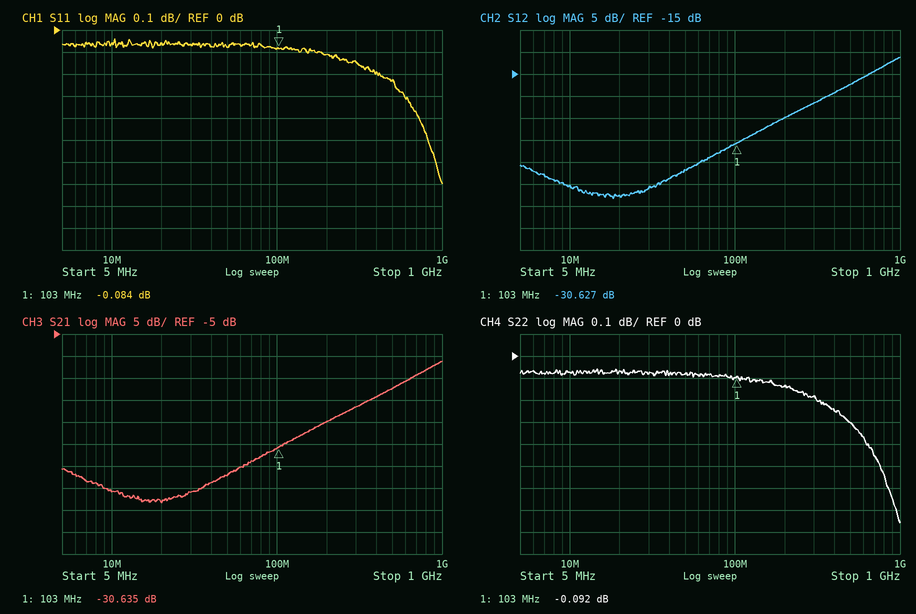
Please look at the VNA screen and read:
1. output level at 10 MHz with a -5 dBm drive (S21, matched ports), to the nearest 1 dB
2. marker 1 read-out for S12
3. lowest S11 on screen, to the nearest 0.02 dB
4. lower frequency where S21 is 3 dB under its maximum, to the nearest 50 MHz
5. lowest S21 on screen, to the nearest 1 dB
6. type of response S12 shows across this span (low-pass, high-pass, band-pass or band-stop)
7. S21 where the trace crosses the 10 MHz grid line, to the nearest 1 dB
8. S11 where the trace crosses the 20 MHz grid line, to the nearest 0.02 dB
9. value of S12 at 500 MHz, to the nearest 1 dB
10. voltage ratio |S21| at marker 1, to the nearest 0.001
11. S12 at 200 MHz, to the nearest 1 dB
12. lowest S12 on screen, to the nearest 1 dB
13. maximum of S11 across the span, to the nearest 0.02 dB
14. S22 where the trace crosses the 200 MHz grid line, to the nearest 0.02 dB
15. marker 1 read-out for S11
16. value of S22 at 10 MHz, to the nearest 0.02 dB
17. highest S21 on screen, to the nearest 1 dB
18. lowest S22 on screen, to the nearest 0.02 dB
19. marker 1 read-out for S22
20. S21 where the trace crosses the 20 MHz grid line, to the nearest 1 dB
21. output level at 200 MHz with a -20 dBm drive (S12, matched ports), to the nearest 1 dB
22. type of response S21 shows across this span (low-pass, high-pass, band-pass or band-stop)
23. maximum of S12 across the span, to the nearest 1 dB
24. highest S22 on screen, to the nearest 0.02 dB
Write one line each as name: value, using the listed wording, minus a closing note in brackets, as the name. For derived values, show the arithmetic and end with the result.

output level at 10 MHz with a -5 dBm drive (S21, matched ports), to the nearest 1 dB: -5 dBm + (-41 dB) = -46 dBm
marker 1 read-out for S12: -30.627 dB
lowest S11 on screen, to the nearest 0.02 dB: -0.70 dB
lower frequency where S21 is 3 dB under its maximum, to the nearest 50 MHz: 700 MHz
lowest S21 on screen, to the nearest 1 dB: -43 dB
type of response S12 shows across this span: high-pass
S21 where the trace crosses the 10 MHz grid line, to the nearest 1 dB: -41 dB
S11 where the trace crosses the 20 MHz grid line, to the nearest 0.02 dB: -0.06 dB
value of S12 at 500 MHz, to the nearest 1 dB: -17 dB
voltage ratio |S21| at marker 1, to the nearest 0.001: 10^(-30.635/20) ≈ 0.029
S12 at 200 MHz, to the nearest 1 dB: -25 dB
lowest S12 on screen, to the nearest 1 dB: -43 dB
maximum of S11 across the span, to the nearest 0.02 dB: -0.04 dB
S22 where the trace crosses the 200 MHz grid line, to the nearest 0.02 dB: -0.14 dB
marker 1 read-out for S11: -0.084 dB
value of S22 at 10 MHz, to the nearest 0.02 dB: -0.08 dB
highest S21 on screen, to the nearest 1 dB: -11 dB
lowest S22 on screen, to the nearest 0.02 dB: -0.76 dB
marker 1 read-out for S22: -0.092 dB
S21 where the trace crosses the 20 MHz grid line, to the nearest 1 dB: -43 dB
output level at 200 MHz with a -20 dBm drive (S12, matched ports), to the nearest 1 dB: -20 dBm + (-25 dB) = -45 dBm
type of response S21 shows across this span: high-pass
maximum of S12 across the span, to the nearest 1 dB: -11 dB
highest S22 on screen, to the nearest 0.02 dB: -0.06 dB
